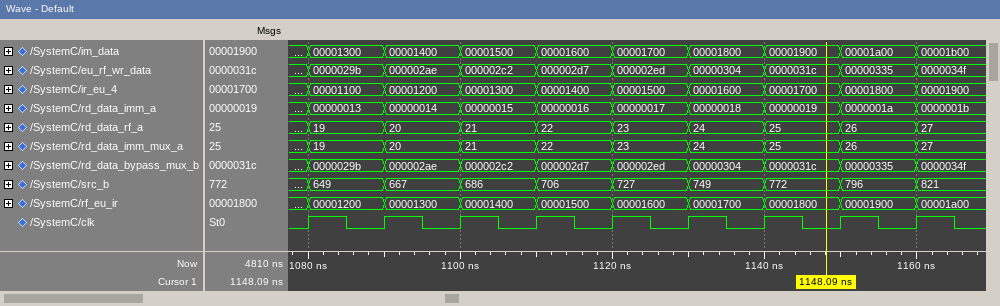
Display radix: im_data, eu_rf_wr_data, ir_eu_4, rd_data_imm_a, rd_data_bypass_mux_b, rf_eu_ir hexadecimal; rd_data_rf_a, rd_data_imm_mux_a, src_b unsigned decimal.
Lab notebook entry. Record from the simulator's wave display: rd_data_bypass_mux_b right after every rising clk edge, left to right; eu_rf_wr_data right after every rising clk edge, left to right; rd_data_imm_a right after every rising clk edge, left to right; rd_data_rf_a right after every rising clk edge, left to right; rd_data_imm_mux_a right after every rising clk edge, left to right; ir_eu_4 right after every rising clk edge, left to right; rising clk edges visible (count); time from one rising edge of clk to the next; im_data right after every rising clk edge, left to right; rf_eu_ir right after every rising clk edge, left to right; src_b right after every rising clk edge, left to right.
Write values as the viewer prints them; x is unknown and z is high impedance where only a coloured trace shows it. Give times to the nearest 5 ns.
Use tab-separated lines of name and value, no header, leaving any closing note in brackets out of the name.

rd_data_bypass_mux_b right after every rising clk edge, left to right	0000029b, 000002ae, 000002c2, 000002d7, 000002ed, 00000304, 0000031c, 00000335, 0000034f
eu_rf_wr_data right after every rising clk edge, left to right	0000029b, 000002ae, 000002c2, 000002d7, 000002ed, 00000304, 0000031c, 00000335, 0000034f
rd_data_imm_a right after every rising clk edge, left to right	00000013, 00000014, 00000015, 00000016, 00000017, 00000018, 00000019, 0000001a, 0000001b
rd_data_rf_a right after every rising clk edge, left to right	19, 20, 21, 22, 23, 24, 25, 26, 27
rd_data_imm_mux_a right after every rising clk edge, left to right	19, 20, 21, 22, 23, 24, 25, 26, 27
ir_eu_4 right after every rising clk edge, left to right	00001100, 00001200, 00001300, 00001400, 00001500, 00001600, 00001700, 00001800, 00001900
rising clk edges visible	9
time from one rising edge of clk to the next	10 ns
im_data right after every rising clk edge, left to right	00001300, 00001400, 00001500, 00001600, 00001700, 00001800, 00001900, 00001a00, 00001b00
rf_eu_ir right after every rising clk edge, left to right	00001200, 00001300, 00001400, 00001500, 00001600, 00001700, 00001800, 00001900, 00001a00
src_b right after every rising clk edge, left to right	649, 667, 686, 706, 727, 749, 772, 796, 821
